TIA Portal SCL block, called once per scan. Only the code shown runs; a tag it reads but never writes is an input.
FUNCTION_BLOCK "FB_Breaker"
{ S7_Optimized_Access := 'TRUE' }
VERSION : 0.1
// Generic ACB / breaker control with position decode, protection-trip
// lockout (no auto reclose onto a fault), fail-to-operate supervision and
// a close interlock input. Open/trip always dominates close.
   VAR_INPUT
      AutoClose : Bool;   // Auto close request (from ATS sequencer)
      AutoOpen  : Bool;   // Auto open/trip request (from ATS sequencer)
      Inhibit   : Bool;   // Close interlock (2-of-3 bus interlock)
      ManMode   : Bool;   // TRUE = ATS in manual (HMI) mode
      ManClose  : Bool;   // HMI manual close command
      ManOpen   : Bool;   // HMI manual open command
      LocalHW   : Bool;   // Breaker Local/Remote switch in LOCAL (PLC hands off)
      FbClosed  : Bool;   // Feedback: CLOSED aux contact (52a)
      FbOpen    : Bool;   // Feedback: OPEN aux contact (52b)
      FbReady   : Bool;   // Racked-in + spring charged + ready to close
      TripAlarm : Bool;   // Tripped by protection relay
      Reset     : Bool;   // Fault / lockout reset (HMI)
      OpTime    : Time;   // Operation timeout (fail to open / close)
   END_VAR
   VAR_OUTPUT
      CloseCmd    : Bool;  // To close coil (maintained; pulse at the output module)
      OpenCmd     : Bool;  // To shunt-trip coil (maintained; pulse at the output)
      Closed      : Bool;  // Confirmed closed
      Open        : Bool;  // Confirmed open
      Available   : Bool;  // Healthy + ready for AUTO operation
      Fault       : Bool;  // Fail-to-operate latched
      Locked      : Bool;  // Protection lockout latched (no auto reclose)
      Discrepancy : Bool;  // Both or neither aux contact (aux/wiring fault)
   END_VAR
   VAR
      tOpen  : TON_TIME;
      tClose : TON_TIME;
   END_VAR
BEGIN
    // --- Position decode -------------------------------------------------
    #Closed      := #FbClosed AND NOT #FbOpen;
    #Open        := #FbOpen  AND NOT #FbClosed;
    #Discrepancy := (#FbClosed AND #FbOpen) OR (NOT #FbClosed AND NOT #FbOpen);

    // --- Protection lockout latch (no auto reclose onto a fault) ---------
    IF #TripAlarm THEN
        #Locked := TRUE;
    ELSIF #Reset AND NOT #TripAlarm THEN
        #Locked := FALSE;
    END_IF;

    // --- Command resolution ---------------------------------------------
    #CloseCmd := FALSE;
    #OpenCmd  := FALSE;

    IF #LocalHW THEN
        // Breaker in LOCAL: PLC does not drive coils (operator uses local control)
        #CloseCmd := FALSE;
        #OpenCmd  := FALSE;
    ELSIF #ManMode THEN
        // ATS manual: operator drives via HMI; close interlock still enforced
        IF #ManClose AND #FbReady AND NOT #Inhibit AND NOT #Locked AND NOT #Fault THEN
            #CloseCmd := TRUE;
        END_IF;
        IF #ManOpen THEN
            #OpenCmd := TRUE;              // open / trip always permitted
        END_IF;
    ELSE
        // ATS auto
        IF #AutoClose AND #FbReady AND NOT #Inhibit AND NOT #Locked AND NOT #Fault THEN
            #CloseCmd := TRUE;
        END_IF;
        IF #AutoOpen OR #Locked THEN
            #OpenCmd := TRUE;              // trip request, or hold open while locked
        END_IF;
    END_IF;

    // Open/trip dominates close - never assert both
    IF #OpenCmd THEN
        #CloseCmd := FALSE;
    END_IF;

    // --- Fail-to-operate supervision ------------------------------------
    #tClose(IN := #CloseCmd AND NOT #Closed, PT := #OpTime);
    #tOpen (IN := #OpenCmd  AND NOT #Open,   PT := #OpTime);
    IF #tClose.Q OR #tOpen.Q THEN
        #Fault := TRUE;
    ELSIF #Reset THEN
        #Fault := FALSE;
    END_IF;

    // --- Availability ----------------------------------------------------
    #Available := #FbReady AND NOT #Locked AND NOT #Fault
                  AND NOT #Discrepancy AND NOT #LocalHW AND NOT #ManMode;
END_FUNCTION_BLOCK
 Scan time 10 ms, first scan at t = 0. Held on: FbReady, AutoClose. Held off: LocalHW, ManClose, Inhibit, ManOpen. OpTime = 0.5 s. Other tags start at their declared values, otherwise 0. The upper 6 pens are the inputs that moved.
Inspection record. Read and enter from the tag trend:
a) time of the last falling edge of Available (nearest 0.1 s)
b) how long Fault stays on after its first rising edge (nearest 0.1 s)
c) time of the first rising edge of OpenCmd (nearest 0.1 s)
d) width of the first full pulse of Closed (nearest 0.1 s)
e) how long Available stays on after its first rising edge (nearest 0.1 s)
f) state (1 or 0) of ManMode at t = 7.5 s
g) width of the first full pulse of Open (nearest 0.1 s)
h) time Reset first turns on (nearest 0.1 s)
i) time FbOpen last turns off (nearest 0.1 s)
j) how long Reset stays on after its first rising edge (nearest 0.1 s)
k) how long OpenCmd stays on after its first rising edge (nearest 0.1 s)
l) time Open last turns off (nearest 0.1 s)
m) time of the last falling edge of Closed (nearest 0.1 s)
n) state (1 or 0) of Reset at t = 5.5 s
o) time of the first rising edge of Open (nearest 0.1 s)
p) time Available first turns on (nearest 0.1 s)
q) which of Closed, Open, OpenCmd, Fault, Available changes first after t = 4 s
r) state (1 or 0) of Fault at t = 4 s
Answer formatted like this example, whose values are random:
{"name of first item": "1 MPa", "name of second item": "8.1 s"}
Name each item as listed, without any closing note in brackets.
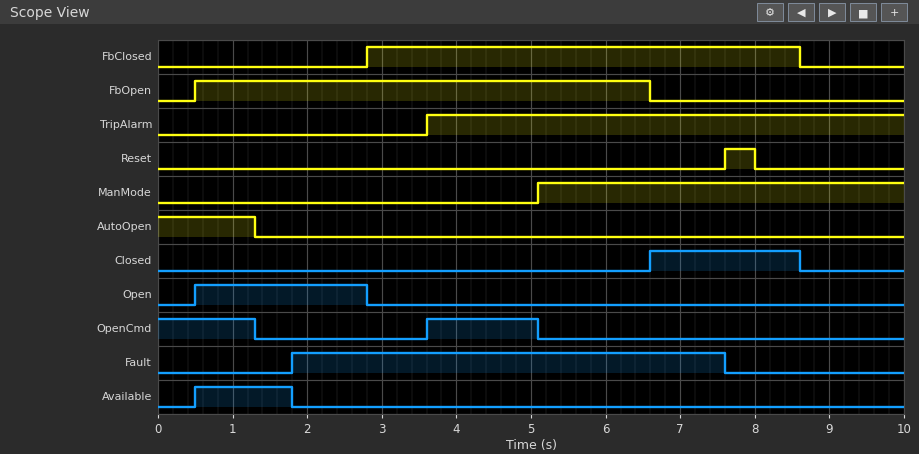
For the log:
{"time of the last falling edge of Available": "1.8 s", "how long Fault stays on after its first rising edge": "5.8 s", "time of the first rising edge of OpenCmd": "3.6 s", "width of the first full pulse of Closed": "2.0 s", "how long Available stays on after its first rising edge": "1.3 s", "state (1 or 0) of ManMode at t = 7.5 s": "1", "width of the first full pulse of Open": "2.3 s", "time Reset first turns on": "7.6 s", "time FbOpen last turns off": "6.6 s", "how long Reset stays on after its first rising edge": "0.4 s", "how long OpenCmd stays on after its first rising edge": "1.5 s", "time Open last turns off": "2.8 s", "time of the last falling edge of Closed": "8.6 s", "state (1 or 0) of Reset at t = 5.5 s": "0", "time of the first rising edge of Open": "0.5 s", "time Available first turns on": "0.5 s", "which of Closed, Open, OpenCmd, Fault, Available changes first after t = 4 s": "OpenCmd", "state (1 or 0) of Fault at t = 4 s": "1"}
